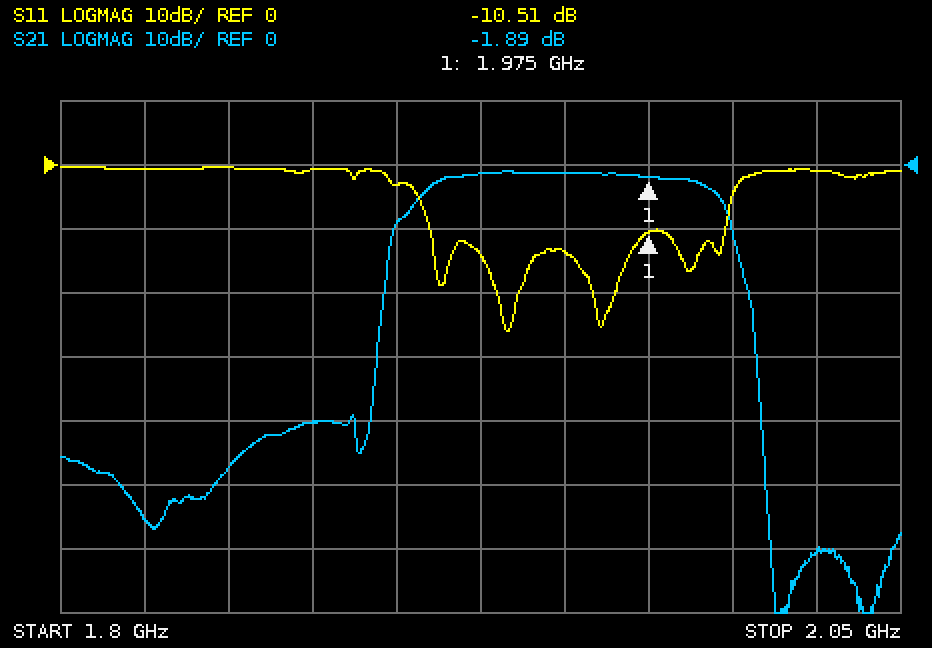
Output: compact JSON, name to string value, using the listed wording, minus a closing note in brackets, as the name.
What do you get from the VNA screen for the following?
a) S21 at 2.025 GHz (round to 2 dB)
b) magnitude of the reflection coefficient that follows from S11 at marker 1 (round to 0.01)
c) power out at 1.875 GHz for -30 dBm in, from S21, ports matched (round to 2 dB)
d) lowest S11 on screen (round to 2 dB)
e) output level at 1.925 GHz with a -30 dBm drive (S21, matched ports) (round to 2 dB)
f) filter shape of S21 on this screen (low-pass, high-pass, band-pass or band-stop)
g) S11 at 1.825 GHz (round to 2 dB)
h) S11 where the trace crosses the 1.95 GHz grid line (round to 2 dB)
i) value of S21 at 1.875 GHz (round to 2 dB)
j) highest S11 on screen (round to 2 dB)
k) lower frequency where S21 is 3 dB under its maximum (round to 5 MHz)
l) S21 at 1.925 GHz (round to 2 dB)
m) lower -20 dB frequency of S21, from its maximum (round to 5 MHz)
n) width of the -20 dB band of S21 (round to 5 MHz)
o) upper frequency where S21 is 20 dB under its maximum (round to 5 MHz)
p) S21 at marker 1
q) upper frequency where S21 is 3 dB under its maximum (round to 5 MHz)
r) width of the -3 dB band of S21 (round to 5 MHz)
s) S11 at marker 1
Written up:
{"S21 at 2.025 GHz": "-60 dB", "magnitude of the reflection coefficient that follows from S11 at marker 1": "0.30", "power out at 1.875 GHz for -30 dBm in, from S21, ports matched": "-70 dBm", "lowest S11 on screen": "-26 dB", "output level at 1.925 GHz with a -30 dBm drive (S21, matched ports)": "-32 dBm", "filter shape of S21 on this screen": "band-pass", "S11 at 1.825 GHz": "0 dB", "S11 where the trace crosses the 1.95 GHz grid line": "-14 dB", "value of S21 at 1.875 GHz": "-40 dB", "highest S11 on screen": "0 dB", "lower frequency where S21 is 3 dB under its maximum": "1.910 GHz", "S21 at 1.925 GHz": "-2 dB", "lower -20 dB frequency of S21, from its maximum": "1.895 GHz", "width of the -20 dB band of S21": "110 MHz", "upper frequency where S21 is 20 dB under its maximum": "2.005 GHz", "S21 at marker 1": "-1.89 dB", "upper frequency where S21 is 3 dB under its maximum": "1.995 GHz", "width of the -3 dB band of S21": "85 MHz", "S11 at marker 1": "-10.51 dB"}
